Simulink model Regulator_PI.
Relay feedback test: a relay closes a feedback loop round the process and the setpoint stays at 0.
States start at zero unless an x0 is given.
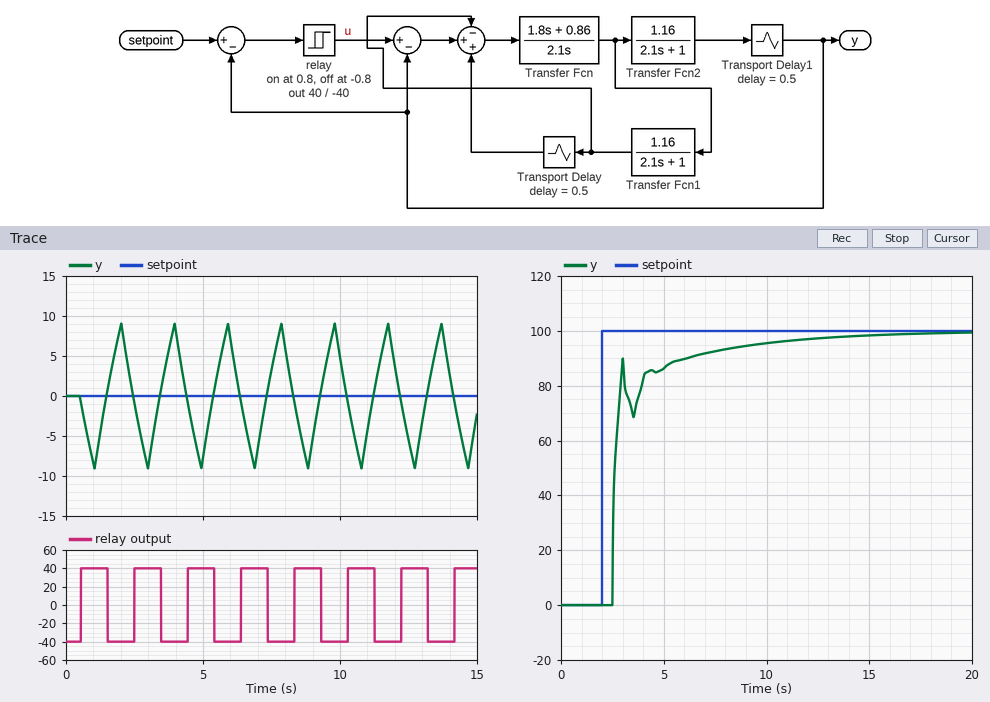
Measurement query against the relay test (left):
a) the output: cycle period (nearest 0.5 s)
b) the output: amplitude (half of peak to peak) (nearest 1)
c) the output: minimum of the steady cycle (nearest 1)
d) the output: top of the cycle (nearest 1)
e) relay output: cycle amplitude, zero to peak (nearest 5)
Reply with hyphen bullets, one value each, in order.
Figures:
- 2.0 s
- 9
- -9
- 9
- 40
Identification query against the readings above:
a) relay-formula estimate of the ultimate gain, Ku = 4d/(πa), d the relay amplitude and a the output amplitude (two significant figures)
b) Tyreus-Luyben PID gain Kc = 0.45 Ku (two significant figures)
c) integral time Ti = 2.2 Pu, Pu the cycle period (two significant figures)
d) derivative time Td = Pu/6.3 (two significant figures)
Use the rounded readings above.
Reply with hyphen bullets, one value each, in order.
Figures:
- 5.7
- 2.6
- 4.4 s
- 0.32 s
